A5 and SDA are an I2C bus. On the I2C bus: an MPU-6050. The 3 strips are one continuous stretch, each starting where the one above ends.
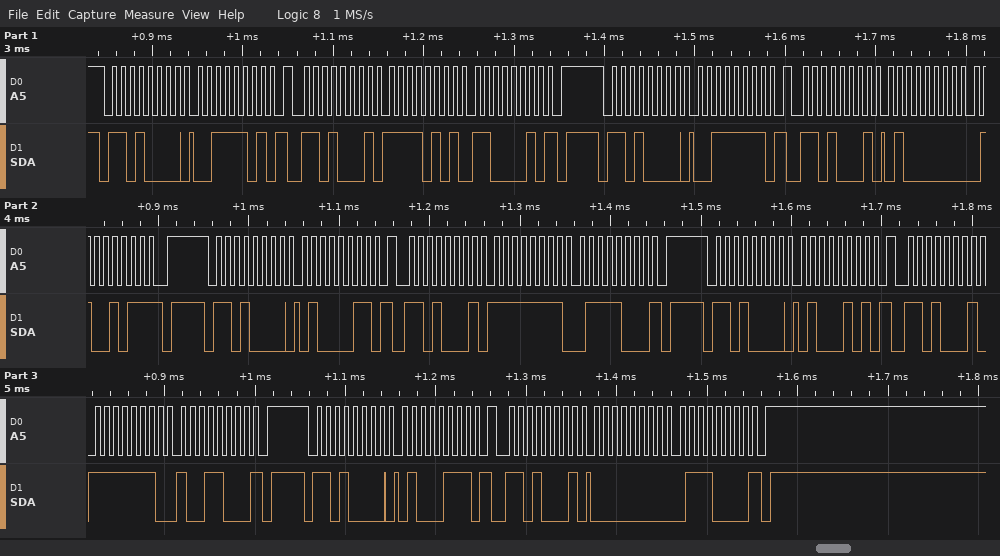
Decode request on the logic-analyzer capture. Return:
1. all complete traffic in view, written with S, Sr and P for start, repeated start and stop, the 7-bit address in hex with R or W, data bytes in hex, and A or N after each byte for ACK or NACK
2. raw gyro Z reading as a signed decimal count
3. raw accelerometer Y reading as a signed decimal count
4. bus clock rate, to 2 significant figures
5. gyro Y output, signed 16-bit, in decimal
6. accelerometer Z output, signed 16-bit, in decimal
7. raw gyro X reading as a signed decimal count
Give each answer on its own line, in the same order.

S 68W A 3D A Sr 68R A F5 A C2 N P S 68W A 3F A Sr 68R A 40 A 4B N P S 68W A 43 A Sr 68R A FF A 78 N P S 68W A 45 A Sr 68R A FE A 98 N P S 68W A 47 A Sr 68R A 00 A 70 N P
112
-2622
100 kHz
-360
16459
-136
